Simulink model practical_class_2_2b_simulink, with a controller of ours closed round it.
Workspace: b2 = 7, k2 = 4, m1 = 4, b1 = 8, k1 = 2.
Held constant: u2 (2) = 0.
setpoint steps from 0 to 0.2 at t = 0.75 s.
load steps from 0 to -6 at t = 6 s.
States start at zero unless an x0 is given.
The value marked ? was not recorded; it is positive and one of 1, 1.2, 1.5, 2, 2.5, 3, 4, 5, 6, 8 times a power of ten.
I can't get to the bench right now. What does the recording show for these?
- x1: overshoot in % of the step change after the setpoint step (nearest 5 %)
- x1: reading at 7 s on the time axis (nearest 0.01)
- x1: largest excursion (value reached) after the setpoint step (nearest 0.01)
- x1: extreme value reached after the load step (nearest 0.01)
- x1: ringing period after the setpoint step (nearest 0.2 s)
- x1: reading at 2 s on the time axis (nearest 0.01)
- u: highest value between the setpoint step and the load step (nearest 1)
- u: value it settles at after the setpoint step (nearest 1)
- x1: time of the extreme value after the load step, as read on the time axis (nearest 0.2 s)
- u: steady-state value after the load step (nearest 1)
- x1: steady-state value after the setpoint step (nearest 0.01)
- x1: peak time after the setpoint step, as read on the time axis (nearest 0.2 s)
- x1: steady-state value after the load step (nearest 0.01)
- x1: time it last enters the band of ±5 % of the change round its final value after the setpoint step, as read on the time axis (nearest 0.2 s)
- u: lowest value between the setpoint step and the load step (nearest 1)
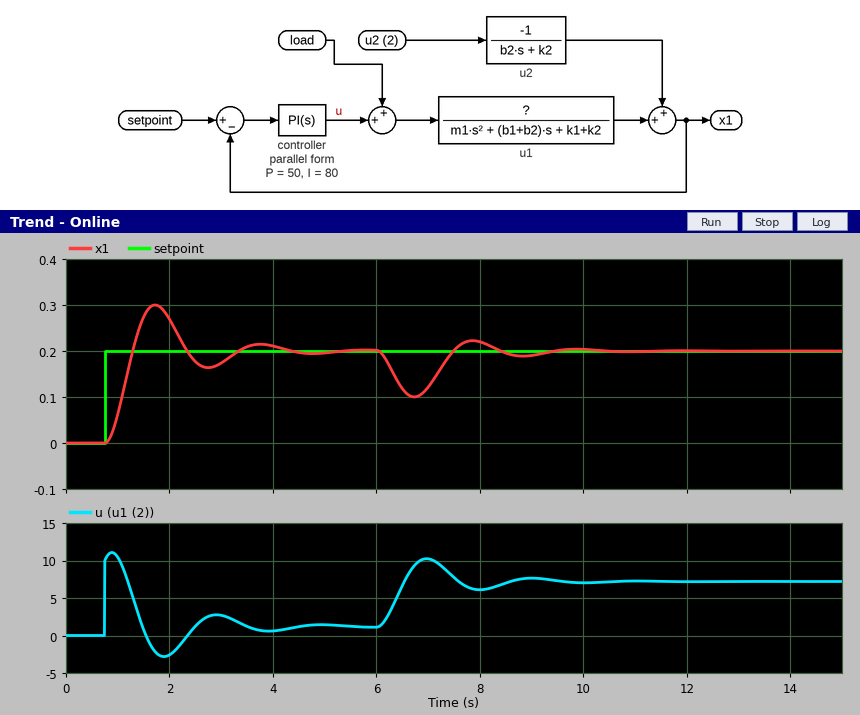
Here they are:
50 %
0.12
0.30
0.10
2.0 s
0.27
11
1
6.8 s
7
0.20
1.8 s
0.20
4.0 s
-3
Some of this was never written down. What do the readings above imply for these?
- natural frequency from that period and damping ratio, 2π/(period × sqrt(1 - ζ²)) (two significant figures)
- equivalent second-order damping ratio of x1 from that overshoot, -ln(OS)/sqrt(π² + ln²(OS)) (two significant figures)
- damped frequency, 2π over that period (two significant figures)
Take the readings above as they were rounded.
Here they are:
3.2 rad/s
0.22
3.1 rad/s
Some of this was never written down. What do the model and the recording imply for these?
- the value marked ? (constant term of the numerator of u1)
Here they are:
1
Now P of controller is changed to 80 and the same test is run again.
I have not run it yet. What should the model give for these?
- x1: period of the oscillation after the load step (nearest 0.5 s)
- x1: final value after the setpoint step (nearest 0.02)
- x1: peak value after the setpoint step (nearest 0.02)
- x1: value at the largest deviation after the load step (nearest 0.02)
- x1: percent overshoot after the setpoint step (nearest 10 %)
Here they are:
1.5 s
0.20
0.28
0.12
40 %
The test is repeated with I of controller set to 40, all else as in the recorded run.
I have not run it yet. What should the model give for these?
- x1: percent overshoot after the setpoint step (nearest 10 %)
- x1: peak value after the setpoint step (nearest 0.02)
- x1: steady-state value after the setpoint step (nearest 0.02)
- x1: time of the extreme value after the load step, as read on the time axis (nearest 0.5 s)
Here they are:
30 %
0.26
0.20
7.0 s
